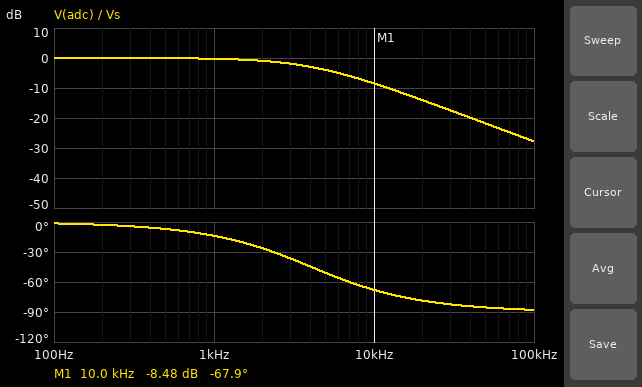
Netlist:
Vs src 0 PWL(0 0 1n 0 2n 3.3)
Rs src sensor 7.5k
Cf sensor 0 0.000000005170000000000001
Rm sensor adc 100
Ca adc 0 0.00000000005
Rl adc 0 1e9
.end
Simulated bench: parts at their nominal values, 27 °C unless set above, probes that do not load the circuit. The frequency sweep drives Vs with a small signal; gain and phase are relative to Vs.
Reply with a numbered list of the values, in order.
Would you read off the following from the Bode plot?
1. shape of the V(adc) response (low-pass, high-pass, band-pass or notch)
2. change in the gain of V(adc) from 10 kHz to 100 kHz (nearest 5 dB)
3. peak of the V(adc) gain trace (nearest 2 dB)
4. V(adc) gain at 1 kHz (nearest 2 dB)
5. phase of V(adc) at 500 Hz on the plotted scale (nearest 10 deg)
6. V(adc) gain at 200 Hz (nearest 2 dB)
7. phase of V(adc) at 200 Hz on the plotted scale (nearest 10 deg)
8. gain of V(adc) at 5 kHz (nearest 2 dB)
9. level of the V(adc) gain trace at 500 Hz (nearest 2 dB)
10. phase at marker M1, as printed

1. low-pass
2. -20 dB
3. 0 dB
4. 0 dB
5. -10 deg
6. 0 dB
7. 0 deg
8. -4 dB
9. 0 dB
10. -67.9 deg
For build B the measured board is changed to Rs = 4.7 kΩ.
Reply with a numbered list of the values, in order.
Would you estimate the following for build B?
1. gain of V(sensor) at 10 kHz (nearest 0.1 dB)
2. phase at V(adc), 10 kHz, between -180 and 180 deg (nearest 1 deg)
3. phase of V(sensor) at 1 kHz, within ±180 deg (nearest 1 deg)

1. -5.3 dB
2. -57 deg
3. -9 deg
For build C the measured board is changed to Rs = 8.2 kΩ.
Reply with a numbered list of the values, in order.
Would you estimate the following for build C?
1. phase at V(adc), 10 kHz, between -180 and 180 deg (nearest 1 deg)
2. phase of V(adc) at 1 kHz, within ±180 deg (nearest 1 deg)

1. -70 deg
2. -15 deg
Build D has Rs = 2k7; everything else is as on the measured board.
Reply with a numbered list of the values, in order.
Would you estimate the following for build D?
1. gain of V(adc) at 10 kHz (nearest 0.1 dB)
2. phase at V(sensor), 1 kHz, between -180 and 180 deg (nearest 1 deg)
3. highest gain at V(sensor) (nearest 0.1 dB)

1. -2.5 dB
2. -5 deg
3. 0 dB
